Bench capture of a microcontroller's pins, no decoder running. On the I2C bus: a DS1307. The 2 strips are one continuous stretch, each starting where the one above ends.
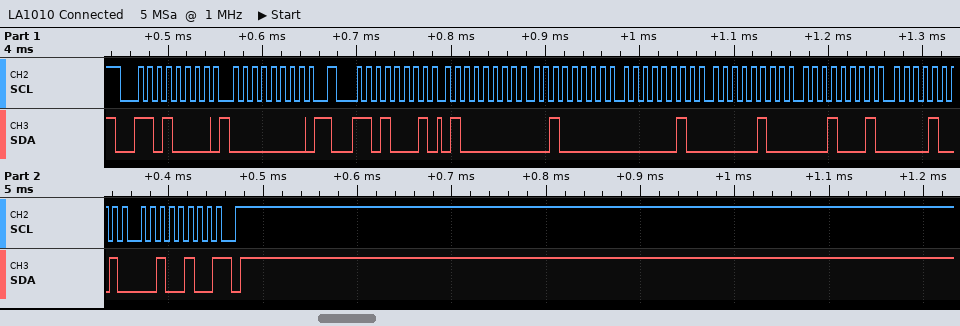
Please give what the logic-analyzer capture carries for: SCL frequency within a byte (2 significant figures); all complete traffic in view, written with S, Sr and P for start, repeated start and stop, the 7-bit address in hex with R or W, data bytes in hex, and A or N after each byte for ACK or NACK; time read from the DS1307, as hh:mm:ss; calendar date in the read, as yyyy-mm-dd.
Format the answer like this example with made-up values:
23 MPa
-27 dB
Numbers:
100 kHz
S 68W A 00 A Sr 68R A 40 A 20 A 02 A 04 A 11 A 09 A 24 N P
02:20:40
2024-09-11
